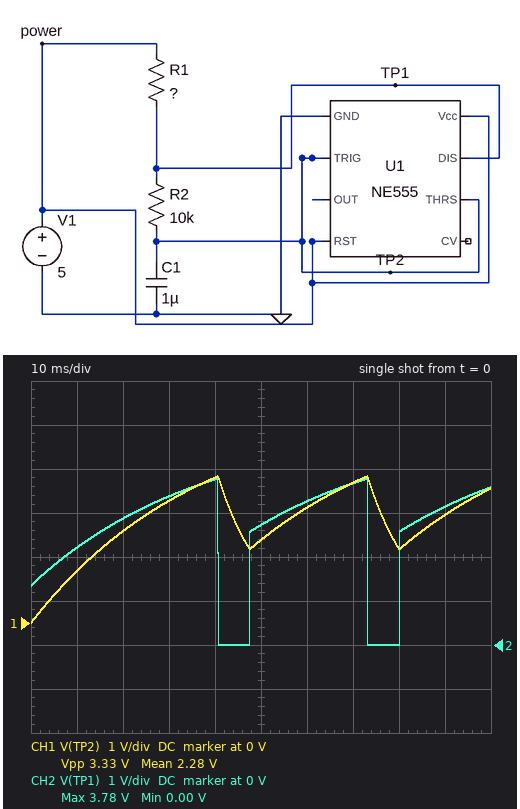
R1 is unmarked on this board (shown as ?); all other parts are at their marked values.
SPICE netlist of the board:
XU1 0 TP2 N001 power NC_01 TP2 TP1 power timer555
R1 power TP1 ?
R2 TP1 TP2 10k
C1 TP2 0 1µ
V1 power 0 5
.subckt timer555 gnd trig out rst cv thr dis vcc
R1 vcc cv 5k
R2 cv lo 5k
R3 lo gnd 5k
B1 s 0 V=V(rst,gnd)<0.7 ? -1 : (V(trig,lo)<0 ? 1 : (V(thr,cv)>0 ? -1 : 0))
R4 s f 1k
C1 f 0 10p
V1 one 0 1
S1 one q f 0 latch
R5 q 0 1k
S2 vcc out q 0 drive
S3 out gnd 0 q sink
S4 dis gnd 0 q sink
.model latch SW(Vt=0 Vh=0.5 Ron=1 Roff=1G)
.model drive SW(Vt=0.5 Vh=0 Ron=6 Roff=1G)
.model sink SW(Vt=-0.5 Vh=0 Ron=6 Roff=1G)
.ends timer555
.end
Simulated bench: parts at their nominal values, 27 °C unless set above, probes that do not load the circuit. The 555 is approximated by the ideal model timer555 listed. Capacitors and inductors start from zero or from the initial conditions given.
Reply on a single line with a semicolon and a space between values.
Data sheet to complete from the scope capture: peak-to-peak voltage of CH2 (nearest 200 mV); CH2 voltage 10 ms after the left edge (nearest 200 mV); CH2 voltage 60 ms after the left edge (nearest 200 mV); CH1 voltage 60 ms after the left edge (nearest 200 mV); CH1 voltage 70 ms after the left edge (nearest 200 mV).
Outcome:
3.8 V; 2.2 V; 3.2 V; 2.6 V; 3.2 V
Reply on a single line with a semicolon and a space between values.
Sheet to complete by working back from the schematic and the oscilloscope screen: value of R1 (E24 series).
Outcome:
27 kΩ
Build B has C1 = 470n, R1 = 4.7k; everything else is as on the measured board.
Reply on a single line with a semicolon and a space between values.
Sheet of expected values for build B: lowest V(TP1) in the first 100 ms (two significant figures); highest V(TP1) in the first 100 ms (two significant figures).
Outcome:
7.4 mV; 4.5 V
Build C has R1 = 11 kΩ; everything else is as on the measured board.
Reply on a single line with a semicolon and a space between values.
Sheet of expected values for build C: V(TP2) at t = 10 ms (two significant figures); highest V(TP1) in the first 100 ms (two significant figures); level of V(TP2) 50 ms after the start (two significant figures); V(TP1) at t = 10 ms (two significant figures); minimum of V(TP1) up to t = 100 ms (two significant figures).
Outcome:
1.9 V; 4.1 V; 1.9 V; 3.4 V; 3.7 mV
